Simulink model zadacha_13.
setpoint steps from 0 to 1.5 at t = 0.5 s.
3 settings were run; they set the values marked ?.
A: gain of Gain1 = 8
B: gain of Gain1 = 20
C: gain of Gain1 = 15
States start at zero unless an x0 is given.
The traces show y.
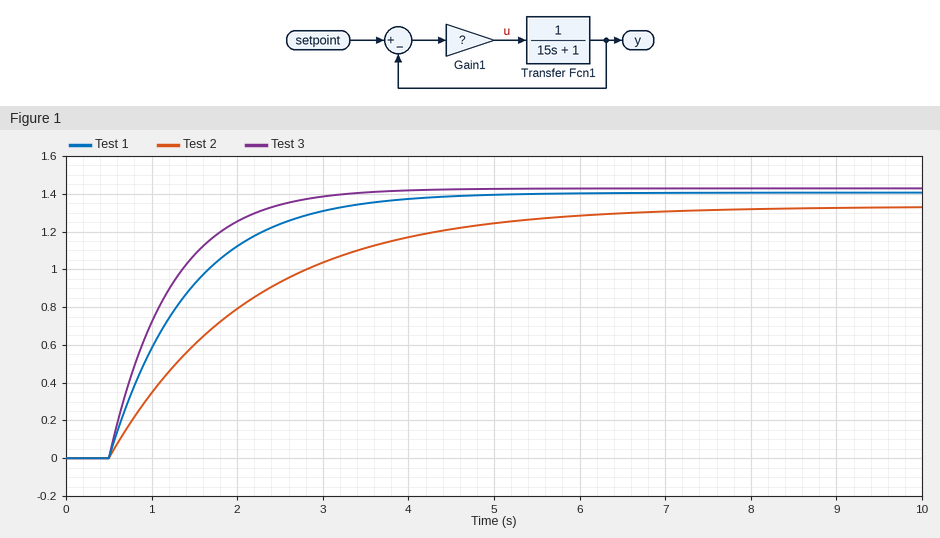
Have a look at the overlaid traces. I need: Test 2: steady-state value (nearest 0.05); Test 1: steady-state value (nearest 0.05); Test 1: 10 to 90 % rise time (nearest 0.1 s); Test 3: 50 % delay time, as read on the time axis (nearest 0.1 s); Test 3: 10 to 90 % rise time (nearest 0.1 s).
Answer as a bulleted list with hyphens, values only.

- 1.35
- 1.40
- 2.1 s
- 1.0 s
- 1.6 s
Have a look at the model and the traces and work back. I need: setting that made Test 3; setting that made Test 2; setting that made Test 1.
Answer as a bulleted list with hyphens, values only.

- B
- A
- C
